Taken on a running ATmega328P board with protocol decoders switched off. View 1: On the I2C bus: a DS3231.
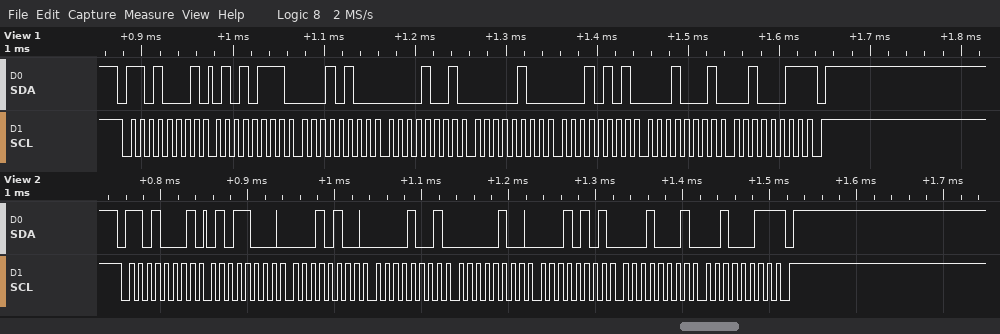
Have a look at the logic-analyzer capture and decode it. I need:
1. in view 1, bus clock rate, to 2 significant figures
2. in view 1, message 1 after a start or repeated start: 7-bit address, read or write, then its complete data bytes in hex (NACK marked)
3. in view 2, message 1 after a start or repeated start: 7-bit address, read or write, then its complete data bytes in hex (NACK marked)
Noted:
100 kHz
0x68 read: 57 14 09 04 15 11 23 NACK
0x68 read: 58 14 09 04 15 11 23 NACK
